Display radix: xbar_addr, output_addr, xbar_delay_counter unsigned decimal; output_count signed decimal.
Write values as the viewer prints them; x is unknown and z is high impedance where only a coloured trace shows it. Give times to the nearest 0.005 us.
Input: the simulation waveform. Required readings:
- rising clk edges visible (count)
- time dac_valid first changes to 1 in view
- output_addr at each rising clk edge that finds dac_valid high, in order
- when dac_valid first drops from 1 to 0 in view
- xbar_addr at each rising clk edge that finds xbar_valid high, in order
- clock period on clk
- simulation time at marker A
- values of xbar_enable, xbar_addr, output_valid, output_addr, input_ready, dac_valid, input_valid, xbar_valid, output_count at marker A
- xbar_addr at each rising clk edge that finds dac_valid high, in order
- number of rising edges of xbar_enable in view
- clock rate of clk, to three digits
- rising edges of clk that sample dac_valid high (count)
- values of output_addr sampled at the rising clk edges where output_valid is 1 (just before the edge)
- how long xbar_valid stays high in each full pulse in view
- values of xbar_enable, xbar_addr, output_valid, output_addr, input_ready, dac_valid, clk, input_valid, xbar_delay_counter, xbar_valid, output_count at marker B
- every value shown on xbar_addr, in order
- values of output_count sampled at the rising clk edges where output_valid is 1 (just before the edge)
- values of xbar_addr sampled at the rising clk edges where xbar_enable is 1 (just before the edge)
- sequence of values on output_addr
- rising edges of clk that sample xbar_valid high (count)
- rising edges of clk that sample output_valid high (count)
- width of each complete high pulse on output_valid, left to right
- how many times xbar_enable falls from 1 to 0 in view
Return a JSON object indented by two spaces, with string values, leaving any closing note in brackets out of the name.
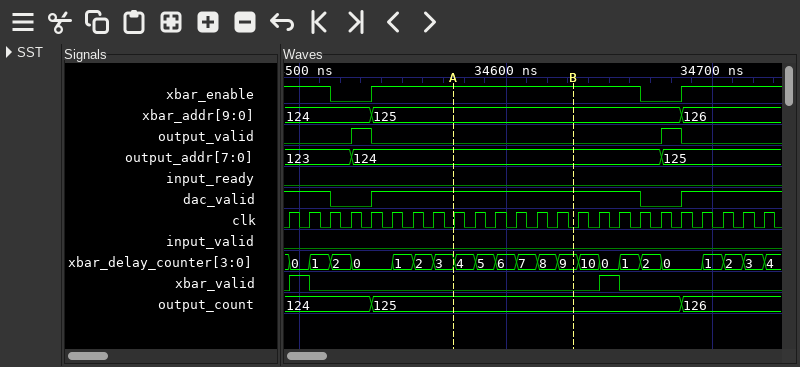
{
  "rising clk edges visible": "24",
  "time dac_valid first changes to 1 in view": "34.535 us",
  "output_addr at each rising clk edge that finds dac_valid high, in order": "123, 123, 123, 124, 124, 124, 124, 124, 124, 124, 124, 124, 124, 124, 124, 124, 125, 125, 125, 125",
  "when dac_valid first drops from 1 to 0 in view": "34.515 us",
  "xbar_addr at each rising clk edge that finds xbar_valid high, in order": "124, 125",
  "clock period on clk": "0.01 us",
  "simulation time at marker A": "34.575 us",
  "values of xbar_enable, xbar_addr, output_valid, output_addr, input_ready, dac_valid, input_valid, xbar_valid, output_count at marker A": "xbar_enable=1, xbar_addr=125, output_valid=0, output_addr=124, input_ready=0, dac_valid=1, input_valid=0, xbar_valid=0, output_count=125",
  "xbar_addr at each rising clk edge that finds dac_valid high, in order": "124, 124, 124, 125, 125, 125, 125, 125, 125, 125, 125, 125, 125, 125, 125, 125, 126, 126, 126, 126",
  "number of rising edges of xbar_enable in view": "2",
  "clock rate of clk, to three digits": "100 MHz",
  "rising edges of clk that sample dac_valid high": "20",
  "values of output_addr sampled at the rising clk edges where output_valid is 1": "124, 125",
  "how long xbar_valid stays high in each full pulse in view": "0.01 us, 0.01 us",
  "values of xbar_enable, xbar_addr, output_valid, output_addr, input_ready, dac_valid, clk, input_valid, xbar_delay_counter, xbar_valid, output_count at marker B": "xbar_enable=1, xbar_addr=125, output_valid=0, output_addr=124, input_ready=0, dac_valid=1, clk=0, input_valid=0, xbar_delay_counter=9, xbar_valid=0, output_count=125",
  "every value shown on xbar_addr, in order": "124, 125, 126",
  "values of output_count sampled at the rising clk edges where output_valid is 1": "124, 125",
  "values of xbar_addr sampled at the rising clk edges where xbar_enable is 1": "124, 124, 124, 125, 125, 125, 125, 125, 125, 125, 125, 125, 125, 125, 125, 125, 126, 126, 126, 126",
  "sequence of values on output_addr": "123, 124, 125",
  "rising edges of clk that sample xbar_valid high": "2",
  "rising edges of clk that sample output_valid high": "2",
  "width of each complete high pulse on output_valid, left to right": "0.01 us, 0.01 us",
  "how many times xbar_enable falls from 1 to 0 in view": "2"
}
